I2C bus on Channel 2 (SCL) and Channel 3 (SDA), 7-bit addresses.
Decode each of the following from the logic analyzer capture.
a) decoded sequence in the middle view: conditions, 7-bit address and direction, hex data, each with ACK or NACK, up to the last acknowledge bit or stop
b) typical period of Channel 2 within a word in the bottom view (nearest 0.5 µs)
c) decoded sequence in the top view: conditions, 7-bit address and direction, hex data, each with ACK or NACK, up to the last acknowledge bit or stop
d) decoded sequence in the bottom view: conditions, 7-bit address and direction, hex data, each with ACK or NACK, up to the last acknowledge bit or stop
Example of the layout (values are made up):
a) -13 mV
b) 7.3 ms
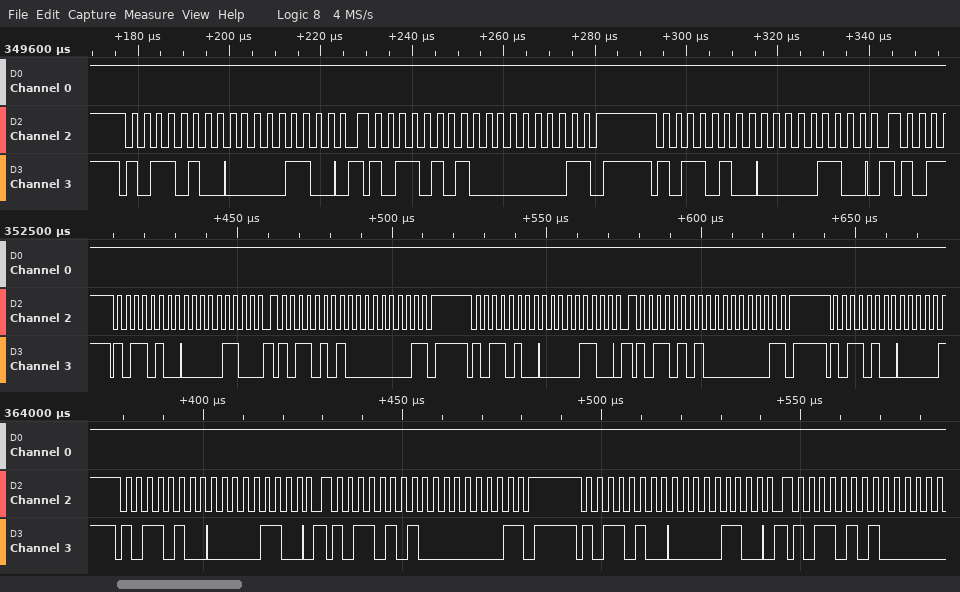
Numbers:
a) start, address 5A write ACK, 0C ACK, repeated start, address 5A read ACK, 01 NACK, stop, start, address 5A write ACK, 0C ACK, repeated start, address 5A read ACK, 01 NACK, stop, start, address 5A write ACK
b) 2.5 µs
c) start, address 5A write ACK, 0C ACK, repeated start, address 5A read ACK, 01 NACK, stop, start, address 5A write ACK, 0C ACK
d) start, address 5A write ACK, 0C ACK, repeated start, address 5A read ACK, 01 NACK, stop, start, address 5A write ACK, 0C ACK, repeated start, address 5A read ACK
